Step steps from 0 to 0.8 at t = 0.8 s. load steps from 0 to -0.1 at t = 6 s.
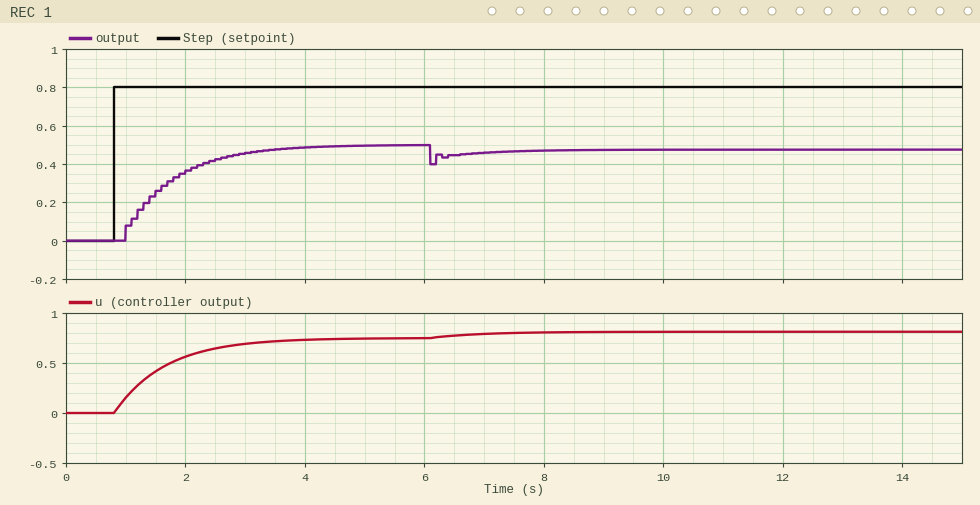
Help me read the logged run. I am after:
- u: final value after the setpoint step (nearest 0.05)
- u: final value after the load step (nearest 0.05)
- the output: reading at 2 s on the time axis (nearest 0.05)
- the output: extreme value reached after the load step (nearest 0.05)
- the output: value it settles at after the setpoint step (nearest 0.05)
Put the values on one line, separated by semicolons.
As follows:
0.75; 0.80; 0.35; 0.40; 0.50
